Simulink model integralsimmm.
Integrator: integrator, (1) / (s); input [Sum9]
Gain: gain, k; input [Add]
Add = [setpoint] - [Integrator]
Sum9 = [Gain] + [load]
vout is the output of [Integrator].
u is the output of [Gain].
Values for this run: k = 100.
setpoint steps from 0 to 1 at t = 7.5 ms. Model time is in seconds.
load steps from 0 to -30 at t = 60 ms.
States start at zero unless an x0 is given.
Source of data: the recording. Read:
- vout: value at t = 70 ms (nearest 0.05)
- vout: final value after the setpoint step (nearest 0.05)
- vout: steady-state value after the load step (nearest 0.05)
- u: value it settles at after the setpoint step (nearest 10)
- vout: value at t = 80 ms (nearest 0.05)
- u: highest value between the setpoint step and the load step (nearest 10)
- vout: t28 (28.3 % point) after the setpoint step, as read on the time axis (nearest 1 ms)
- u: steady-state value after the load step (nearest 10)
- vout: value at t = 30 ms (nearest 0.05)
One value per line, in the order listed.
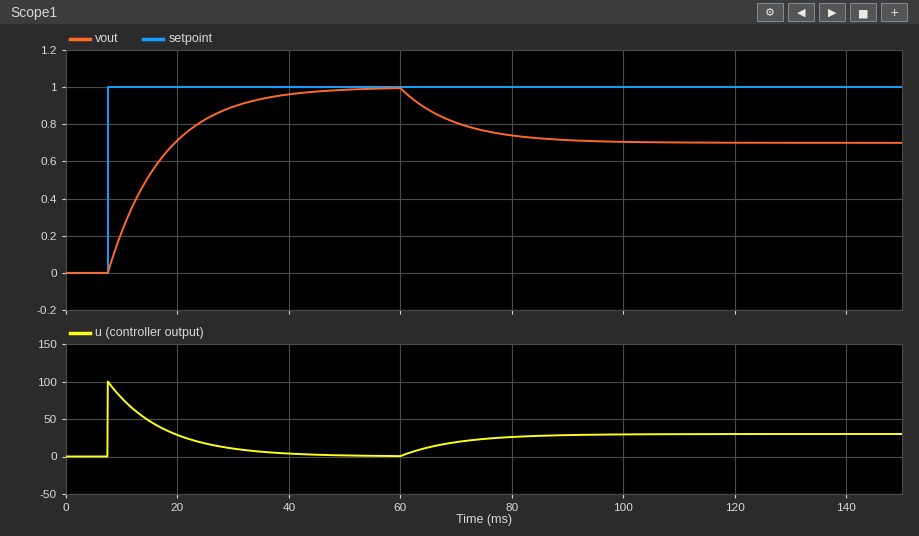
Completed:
0.80
1.00
0.70
0
0.75
100
11 ms
30
0.90
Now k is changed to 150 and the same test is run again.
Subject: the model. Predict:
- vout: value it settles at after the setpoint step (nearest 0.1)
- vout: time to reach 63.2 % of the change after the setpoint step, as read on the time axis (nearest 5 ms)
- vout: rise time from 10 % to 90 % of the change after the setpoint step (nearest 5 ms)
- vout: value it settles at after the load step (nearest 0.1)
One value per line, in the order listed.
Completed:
1.0
15 ms
15 ms
0.8
